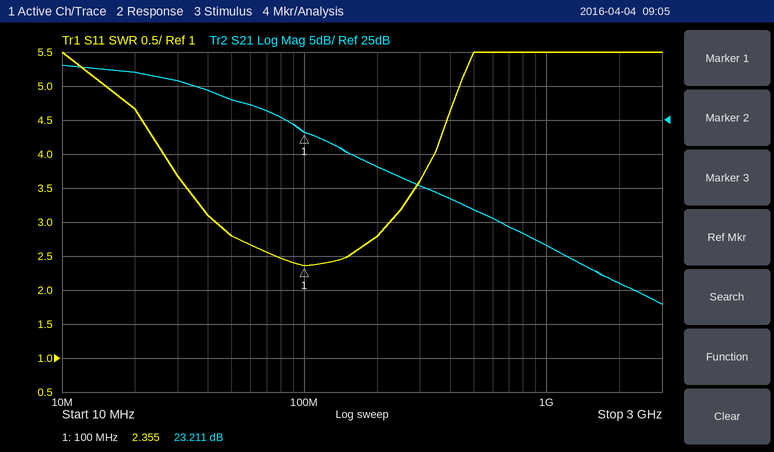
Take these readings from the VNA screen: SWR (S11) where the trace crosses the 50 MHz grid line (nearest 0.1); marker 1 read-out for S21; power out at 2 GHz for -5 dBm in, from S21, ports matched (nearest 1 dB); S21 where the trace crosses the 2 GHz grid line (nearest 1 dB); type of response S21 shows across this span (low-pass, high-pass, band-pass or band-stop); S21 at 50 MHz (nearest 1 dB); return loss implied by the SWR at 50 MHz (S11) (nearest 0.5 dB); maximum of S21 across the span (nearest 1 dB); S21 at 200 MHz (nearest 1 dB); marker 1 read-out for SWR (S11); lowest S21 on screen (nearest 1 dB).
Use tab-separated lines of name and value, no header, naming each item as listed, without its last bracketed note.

SWR (S11) where the trace crosses the 50 MHz grid line	2.8
marker 1 read-out for S21	23.211 dB
power out at 2 GHz for -5 dBm in, from S21, ports matched	-4 dBm
S21 where the trace crosses the 2 GHz grid line	1 dB
type of response S21 shows across this span	low-pass
S21 at 50 MHz	28 dB
return loss implied by the SWR at 50 MHz (S11)	6.5 dB
maximum of S21 across the span	33 dB
S21 at 200 MHz	18 dB
marker 1 read-out for SWR	2.355
lowest S21 on screen	-2 dB
